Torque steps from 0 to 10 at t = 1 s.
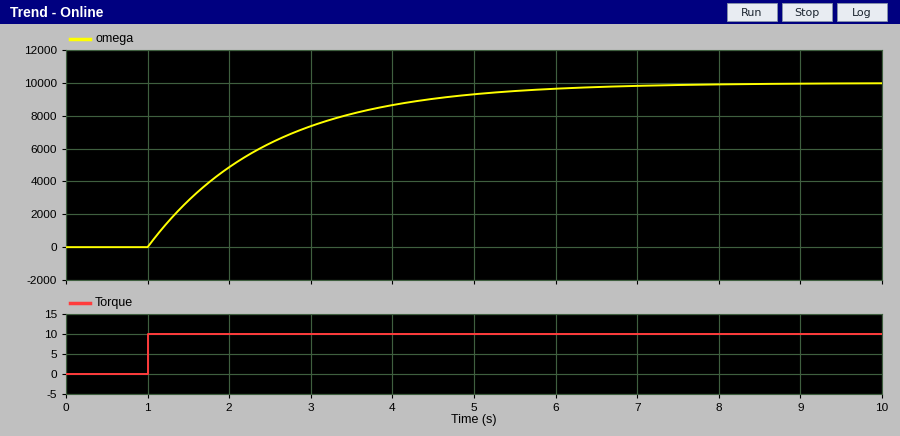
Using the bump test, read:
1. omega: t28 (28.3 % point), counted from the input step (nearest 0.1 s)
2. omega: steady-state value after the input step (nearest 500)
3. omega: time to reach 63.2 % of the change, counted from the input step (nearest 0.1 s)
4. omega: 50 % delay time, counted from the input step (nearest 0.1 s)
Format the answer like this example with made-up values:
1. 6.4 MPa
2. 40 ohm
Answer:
1. 0.5 s
2. 10000
3. 1.5 s
4. 1.0 s
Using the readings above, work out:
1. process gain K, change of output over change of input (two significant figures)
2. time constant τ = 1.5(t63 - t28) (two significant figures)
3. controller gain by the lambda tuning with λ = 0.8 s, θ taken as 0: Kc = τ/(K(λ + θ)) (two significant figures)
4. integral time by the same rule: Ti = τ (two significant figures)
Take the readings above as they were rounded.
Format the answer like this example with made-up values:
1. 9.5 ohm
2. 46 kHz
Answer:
1. 1000
2. 1.5 s
3. 0.0019
4. 1.5 s
